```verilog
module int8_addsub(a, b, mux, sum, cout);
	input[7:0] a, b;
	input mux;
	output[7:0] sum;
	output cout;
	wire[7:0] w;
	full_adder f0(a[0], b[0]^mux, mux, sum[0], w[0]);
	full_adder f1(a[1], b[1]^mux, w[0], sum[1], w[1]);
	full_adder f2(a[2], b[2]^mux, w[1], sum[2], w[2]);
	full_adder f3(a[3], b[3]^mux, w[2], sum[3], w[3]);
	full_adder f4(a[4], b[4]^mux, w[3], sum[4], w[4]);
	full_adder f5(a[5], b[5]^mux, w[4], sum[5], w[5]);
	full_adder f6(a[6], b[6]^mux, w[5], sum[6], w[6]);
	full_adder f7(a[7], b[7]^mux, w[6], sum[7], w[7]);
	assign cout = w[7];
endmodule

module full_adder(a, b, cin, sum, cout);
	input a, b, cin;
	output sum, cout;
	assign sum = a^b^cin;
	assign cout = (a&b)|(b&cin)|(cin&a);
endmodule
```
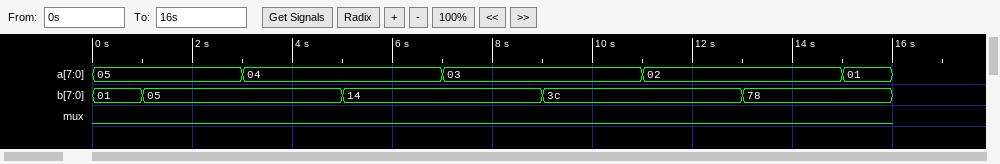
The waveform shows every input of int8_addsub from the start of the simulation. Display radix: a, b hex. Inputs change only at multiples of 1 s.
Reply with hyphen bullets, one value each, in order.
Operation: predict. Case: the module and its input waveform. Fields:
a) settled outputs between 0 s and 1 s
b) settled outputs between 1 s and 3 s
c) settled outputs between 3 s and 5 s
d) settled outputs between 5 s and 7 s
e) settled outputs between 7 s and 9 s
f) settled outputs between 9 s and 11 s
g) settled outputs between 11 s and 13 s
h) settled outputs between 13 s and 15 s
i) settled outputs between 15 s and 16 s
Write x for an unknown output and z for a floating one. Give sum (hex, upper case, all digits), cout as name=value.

- sum=06, cout=0
- sum=0A, cout=0
- sum=09, cout=0
- sum=18, cout=0
- sum=17, cout=0
- sum=3F, cout=0
- sum=3E, cout=0
- sum=7A, cout=0
- sum=79, cout=0
